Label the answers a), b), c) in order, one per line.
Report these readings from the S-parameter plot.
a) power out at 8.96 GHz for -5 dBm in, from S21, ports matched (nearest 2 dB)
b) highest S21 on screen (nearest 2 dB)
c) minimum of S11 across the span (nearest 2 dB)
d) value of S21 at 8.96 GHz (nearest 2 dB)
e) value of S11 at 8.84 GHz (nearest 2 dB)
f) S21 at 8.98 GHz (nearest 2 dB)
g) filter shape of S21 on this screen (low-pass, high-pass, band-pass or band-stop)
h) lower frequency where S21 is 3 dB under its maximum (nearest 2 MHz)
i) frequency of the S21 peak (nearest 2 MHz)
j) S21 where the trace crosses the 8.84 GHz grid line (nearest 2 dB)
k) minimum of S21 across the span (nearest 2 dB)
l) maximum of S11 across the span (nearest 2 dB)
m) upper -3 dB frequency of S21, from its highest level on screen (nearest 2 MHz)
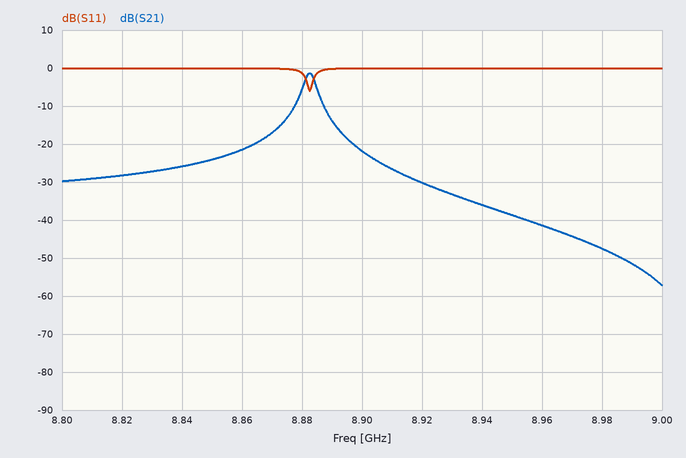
a) -46 dBm
b) -2 dB
c) -6 dB
d) -42 dB
e) 0 dB
f) -48 dB
g) band-pass
h) 8.880 GHz
i) 8.882 GHz
j) -26 dB
k) -58 dB
l) 0 dB
m) 8.884 GHz
